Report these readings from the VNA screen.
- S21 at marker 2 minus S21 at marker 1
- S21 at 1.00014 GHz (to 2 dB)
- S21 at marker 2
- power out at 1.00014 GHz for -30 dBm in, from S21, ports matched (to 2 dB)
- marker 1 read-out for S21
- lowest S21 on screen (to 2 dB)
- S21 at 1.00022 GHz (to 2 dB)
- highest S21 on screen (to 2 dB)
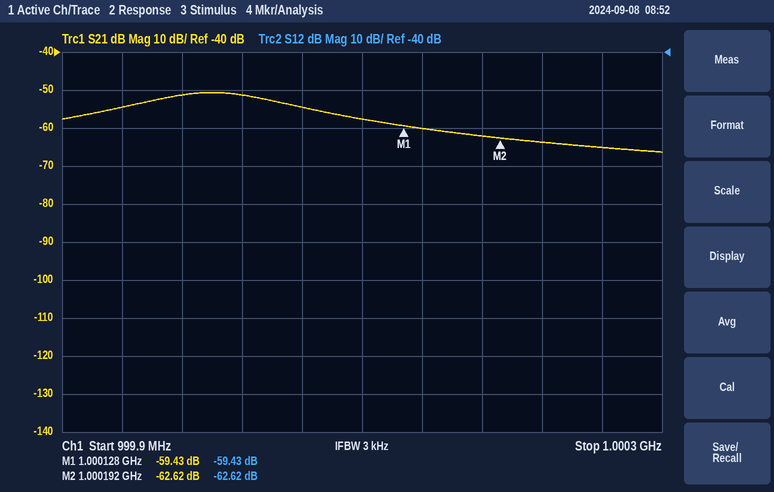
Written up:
-3.19 dB
-60 dB
-62.62 dB
-90 dBm
-59.43 dB
-66 dB
-64 dB
-50 dB
